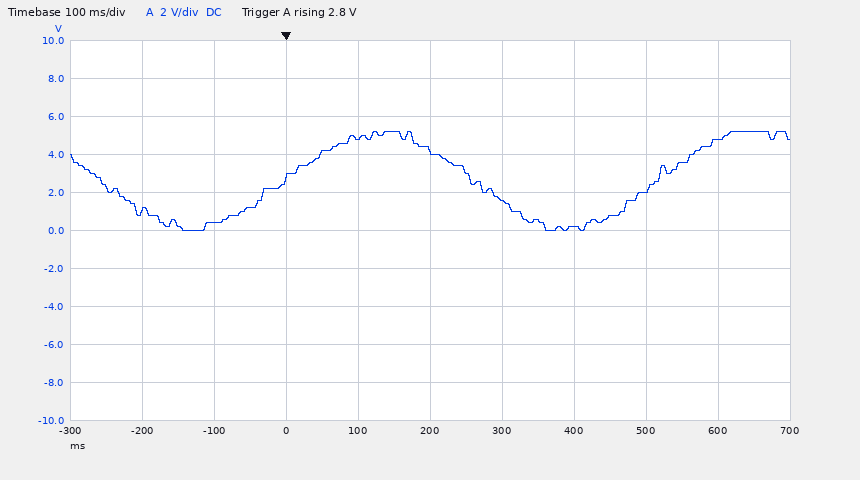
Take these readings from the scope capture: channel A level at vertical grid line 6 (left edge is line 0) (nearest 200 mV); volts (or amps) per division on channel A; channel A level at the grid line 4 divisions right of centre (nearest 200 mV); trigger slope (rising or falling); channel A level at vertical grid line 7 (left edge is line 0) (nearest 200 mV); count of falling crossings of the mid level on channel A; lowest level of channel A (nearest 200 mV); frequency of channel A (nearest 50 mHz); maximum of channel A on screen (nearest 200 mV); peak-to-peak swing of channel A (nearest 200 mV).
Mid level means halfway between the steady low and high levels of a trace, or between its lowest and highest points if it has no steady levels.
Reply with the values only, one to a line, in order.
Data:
1.6 V
2 V
4.8 V
rising
200 mV
2
0.0 V
1.95 Hz
5.2 V
5.2 V
